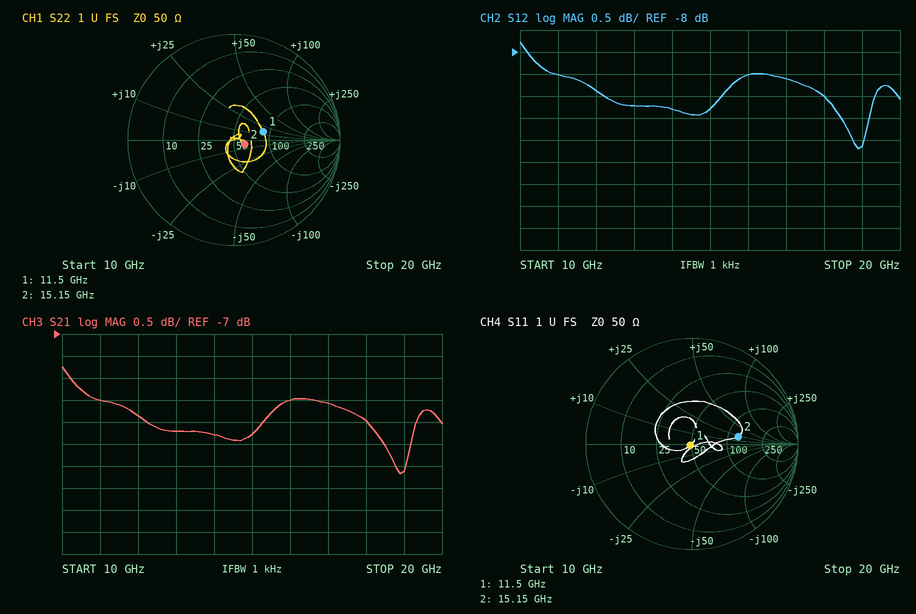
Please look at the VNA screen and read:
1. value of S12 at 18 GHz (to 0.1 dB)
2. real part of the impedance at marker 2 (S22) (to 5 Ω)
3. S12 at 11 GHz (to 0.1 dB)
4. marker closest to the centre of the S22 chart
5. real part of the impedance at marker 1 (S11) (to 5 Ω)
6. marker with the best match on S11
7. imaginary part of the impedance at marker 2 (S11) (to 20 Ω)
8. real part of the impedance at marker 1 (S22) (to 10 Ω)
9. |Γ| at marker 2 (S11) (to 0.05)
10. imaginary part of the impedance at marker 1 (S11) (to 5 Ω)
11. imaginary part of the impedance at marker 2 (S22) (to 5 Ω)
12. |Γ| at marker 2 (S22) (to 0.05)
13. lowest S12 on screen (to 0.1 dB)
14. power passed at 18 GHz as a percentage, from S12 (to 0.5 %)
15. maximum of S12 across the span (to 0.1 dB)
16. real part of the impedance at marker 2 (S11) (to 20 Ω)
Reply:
-9.0 dB
60 Ω
-8.5 dB
marker 2
50 Ω
marker 1
+20 Ω
90 Ω
0.45
0 Ω
-5 Ω
0.10
-10.2 dB
12.5 %
-7.8 dB
120 Ω
